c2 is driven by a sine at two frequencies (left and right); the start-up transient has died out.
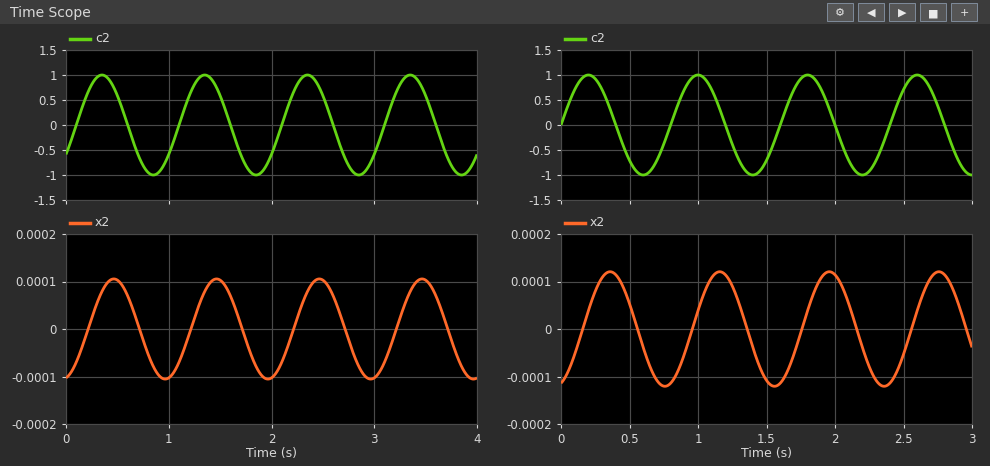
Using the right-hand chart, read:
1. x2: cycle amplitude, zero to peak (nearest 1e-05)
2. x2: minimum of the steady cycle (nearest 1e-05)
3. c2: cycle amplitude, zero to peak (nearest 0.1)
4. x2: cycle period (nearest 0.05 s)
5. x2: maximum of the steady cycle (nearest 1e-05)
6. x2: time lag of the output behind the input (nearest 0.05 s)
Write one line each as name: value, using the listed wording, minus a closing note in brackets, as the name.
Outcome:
x2: cycle amplitude, zero to peak: 0.00012
x2: minimum of the steady cycle: -0.00012
c2: cycle amplitude, zero to peak: 1.0
x2: cycle period: 0.80 s
x2: maximum of the steady cycle: 0.00012
x2: time lag of the output behind the input: 0.15 s
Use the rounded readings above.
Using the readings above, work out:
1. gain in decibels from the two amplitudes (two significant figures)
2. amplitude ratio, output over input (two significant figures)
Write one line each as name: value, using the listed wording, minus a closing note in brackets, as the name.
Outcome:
gain in decibels from the two amplitudes: -78 dB
amplitude ratio, output over input: 0.00012
